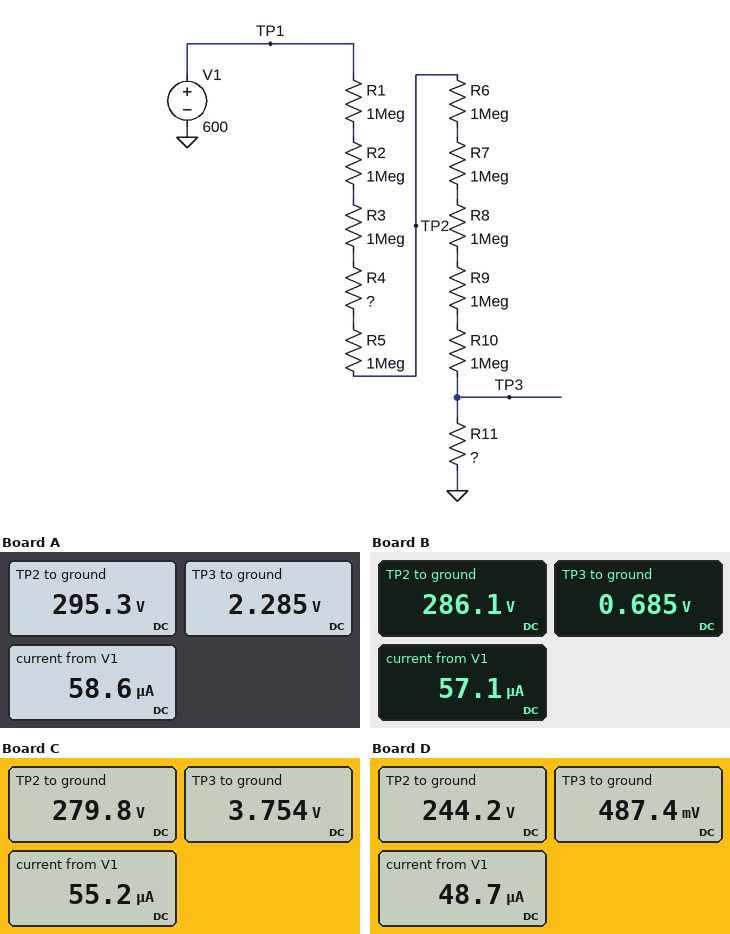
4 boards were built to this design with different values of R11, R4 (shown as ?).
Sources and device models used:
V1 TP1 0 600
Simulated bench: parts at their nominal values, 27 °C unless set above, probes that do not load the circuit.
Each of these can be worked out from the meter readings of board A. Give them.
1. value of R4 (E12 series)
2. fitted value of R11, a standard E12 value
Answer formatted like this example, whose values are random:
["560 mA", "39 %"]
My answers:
["1.2 MΩ", "39 kΩ"]
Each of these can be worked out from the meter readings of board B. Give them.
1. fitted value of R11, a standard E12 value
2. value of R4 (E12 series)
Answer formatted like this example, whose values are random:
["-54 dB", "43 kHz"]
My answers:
["12 kΩ", "1.5 MΩ"]
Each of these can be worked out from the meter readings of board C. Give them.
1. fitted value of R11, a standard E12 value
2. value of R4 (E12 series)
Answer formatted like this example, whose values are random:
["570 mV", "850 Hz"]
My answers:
["68 kΩ", "1.8 MΩ"]
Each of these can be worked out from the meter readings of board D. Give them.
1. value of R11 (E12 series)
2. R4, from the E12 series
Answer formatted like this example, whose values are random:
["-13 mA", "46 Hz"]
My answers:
["10 kΩ", "3.3 MΩ"]
